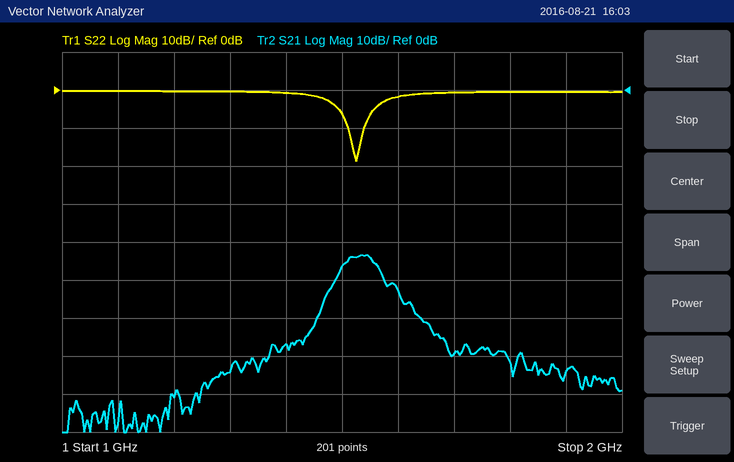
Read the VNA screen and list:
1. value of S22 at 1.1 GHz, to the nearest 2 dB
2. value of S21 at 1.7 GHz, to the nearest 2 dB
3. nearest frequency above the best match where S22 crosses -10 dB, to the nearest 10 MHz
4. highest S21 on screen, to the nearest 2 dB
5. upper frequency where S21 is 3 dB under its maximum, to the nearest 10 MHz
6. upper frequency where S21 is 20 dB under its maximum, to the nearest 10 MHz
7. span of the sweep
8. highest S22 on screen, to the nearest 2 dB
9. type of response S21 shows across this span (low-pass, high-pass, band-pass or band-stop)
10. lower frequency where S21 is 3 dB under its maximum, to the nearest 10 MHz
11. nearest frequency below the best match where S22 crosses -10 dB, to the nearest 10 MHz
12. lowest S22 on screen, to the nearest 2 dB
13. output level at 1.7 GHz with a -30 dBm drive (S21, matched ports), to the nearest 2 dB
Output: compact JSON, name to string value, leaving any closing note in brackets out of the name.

{"value of S22 at 1.1 GHz, to the nearest 2 dB": "0 dB", "value of S21 at 1.7 GHz, to the nearest 2 dB": "-70 dB", "nearest frequency above the best match where S22 crosses -10 dB, to the nearest 10 MHz": "1.54 GHz", "highest S21 on screen, to the nearest 2 dB": "-44 dB", "upper frequency where S21 is 3 dB under its maximum, to the nearest 10 MHz": "1.56 GHz", "upper frequency where S21 is 20 dB under its maximum, to the nearest 10 MHz": "1.66 GHz", "span of the sweep": "1 GHz", "highest S22 on screen, to the nearest 2 dB": "0 dB", "type of response S21 shows across this span": "band-pass", "lower frequency where S21 is 3 dB under its maximum, to the nearest 10 MHz": "1.50 GHz", "nearest frequency below the best match where S22 crosses -10 dB, to the nearest 10 MHz": "1.51 GHz", "lowest S22 on screen, to the nearest 2 dB": "-18 dB", "output level at 1.7 GHz with a -30 dBm drive (S21, matched ports), to the nearest 2 dB": "-100 dBm"}
